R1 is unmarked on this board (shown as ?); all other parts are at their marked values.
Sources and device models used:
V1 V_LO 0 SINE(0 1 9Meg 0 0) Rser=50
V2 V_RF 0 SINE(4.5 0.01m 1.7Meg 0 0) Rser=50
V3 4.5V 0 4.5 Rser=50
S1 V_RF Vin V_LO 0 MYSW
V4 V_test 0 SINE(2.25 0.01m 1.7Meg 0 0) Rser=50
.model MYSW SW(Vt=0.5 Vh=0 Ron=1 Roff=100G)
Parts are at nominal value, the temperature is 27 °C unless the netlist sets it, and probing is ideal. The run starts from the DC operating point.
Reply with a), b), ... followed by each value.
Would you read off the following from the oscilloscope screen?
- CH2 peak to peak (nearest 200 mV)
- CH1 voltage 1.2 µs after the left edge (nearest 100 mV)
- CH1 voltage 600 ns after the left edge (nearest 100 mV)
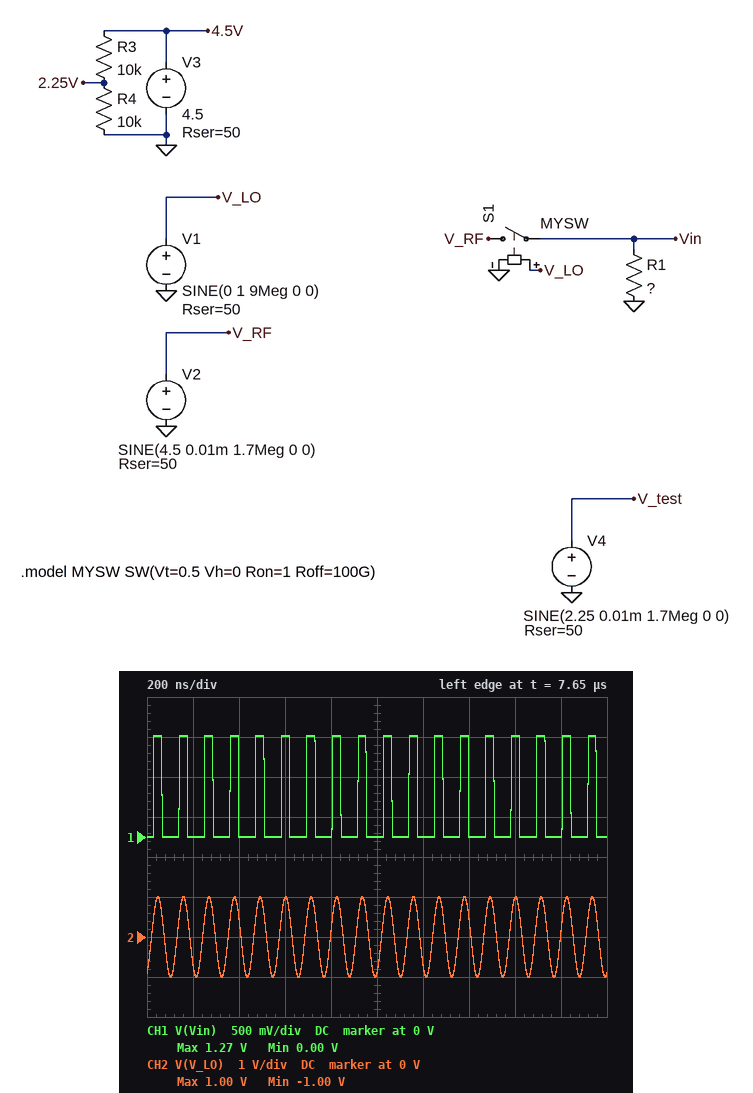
a) 2.0 V
b) 0 V
c) 1.3 V
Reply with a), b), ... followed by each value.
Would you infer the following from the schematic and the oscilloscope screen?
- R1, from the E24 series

a) 20 Ω
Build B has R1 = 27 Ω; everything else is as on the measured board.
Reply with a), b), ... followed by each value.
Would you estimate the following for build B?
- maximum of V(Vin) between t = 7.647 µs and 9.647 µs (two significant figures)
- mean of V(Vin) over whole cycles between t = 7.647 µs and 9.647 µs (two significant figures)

a) 1.6 V
b) 520 mV
